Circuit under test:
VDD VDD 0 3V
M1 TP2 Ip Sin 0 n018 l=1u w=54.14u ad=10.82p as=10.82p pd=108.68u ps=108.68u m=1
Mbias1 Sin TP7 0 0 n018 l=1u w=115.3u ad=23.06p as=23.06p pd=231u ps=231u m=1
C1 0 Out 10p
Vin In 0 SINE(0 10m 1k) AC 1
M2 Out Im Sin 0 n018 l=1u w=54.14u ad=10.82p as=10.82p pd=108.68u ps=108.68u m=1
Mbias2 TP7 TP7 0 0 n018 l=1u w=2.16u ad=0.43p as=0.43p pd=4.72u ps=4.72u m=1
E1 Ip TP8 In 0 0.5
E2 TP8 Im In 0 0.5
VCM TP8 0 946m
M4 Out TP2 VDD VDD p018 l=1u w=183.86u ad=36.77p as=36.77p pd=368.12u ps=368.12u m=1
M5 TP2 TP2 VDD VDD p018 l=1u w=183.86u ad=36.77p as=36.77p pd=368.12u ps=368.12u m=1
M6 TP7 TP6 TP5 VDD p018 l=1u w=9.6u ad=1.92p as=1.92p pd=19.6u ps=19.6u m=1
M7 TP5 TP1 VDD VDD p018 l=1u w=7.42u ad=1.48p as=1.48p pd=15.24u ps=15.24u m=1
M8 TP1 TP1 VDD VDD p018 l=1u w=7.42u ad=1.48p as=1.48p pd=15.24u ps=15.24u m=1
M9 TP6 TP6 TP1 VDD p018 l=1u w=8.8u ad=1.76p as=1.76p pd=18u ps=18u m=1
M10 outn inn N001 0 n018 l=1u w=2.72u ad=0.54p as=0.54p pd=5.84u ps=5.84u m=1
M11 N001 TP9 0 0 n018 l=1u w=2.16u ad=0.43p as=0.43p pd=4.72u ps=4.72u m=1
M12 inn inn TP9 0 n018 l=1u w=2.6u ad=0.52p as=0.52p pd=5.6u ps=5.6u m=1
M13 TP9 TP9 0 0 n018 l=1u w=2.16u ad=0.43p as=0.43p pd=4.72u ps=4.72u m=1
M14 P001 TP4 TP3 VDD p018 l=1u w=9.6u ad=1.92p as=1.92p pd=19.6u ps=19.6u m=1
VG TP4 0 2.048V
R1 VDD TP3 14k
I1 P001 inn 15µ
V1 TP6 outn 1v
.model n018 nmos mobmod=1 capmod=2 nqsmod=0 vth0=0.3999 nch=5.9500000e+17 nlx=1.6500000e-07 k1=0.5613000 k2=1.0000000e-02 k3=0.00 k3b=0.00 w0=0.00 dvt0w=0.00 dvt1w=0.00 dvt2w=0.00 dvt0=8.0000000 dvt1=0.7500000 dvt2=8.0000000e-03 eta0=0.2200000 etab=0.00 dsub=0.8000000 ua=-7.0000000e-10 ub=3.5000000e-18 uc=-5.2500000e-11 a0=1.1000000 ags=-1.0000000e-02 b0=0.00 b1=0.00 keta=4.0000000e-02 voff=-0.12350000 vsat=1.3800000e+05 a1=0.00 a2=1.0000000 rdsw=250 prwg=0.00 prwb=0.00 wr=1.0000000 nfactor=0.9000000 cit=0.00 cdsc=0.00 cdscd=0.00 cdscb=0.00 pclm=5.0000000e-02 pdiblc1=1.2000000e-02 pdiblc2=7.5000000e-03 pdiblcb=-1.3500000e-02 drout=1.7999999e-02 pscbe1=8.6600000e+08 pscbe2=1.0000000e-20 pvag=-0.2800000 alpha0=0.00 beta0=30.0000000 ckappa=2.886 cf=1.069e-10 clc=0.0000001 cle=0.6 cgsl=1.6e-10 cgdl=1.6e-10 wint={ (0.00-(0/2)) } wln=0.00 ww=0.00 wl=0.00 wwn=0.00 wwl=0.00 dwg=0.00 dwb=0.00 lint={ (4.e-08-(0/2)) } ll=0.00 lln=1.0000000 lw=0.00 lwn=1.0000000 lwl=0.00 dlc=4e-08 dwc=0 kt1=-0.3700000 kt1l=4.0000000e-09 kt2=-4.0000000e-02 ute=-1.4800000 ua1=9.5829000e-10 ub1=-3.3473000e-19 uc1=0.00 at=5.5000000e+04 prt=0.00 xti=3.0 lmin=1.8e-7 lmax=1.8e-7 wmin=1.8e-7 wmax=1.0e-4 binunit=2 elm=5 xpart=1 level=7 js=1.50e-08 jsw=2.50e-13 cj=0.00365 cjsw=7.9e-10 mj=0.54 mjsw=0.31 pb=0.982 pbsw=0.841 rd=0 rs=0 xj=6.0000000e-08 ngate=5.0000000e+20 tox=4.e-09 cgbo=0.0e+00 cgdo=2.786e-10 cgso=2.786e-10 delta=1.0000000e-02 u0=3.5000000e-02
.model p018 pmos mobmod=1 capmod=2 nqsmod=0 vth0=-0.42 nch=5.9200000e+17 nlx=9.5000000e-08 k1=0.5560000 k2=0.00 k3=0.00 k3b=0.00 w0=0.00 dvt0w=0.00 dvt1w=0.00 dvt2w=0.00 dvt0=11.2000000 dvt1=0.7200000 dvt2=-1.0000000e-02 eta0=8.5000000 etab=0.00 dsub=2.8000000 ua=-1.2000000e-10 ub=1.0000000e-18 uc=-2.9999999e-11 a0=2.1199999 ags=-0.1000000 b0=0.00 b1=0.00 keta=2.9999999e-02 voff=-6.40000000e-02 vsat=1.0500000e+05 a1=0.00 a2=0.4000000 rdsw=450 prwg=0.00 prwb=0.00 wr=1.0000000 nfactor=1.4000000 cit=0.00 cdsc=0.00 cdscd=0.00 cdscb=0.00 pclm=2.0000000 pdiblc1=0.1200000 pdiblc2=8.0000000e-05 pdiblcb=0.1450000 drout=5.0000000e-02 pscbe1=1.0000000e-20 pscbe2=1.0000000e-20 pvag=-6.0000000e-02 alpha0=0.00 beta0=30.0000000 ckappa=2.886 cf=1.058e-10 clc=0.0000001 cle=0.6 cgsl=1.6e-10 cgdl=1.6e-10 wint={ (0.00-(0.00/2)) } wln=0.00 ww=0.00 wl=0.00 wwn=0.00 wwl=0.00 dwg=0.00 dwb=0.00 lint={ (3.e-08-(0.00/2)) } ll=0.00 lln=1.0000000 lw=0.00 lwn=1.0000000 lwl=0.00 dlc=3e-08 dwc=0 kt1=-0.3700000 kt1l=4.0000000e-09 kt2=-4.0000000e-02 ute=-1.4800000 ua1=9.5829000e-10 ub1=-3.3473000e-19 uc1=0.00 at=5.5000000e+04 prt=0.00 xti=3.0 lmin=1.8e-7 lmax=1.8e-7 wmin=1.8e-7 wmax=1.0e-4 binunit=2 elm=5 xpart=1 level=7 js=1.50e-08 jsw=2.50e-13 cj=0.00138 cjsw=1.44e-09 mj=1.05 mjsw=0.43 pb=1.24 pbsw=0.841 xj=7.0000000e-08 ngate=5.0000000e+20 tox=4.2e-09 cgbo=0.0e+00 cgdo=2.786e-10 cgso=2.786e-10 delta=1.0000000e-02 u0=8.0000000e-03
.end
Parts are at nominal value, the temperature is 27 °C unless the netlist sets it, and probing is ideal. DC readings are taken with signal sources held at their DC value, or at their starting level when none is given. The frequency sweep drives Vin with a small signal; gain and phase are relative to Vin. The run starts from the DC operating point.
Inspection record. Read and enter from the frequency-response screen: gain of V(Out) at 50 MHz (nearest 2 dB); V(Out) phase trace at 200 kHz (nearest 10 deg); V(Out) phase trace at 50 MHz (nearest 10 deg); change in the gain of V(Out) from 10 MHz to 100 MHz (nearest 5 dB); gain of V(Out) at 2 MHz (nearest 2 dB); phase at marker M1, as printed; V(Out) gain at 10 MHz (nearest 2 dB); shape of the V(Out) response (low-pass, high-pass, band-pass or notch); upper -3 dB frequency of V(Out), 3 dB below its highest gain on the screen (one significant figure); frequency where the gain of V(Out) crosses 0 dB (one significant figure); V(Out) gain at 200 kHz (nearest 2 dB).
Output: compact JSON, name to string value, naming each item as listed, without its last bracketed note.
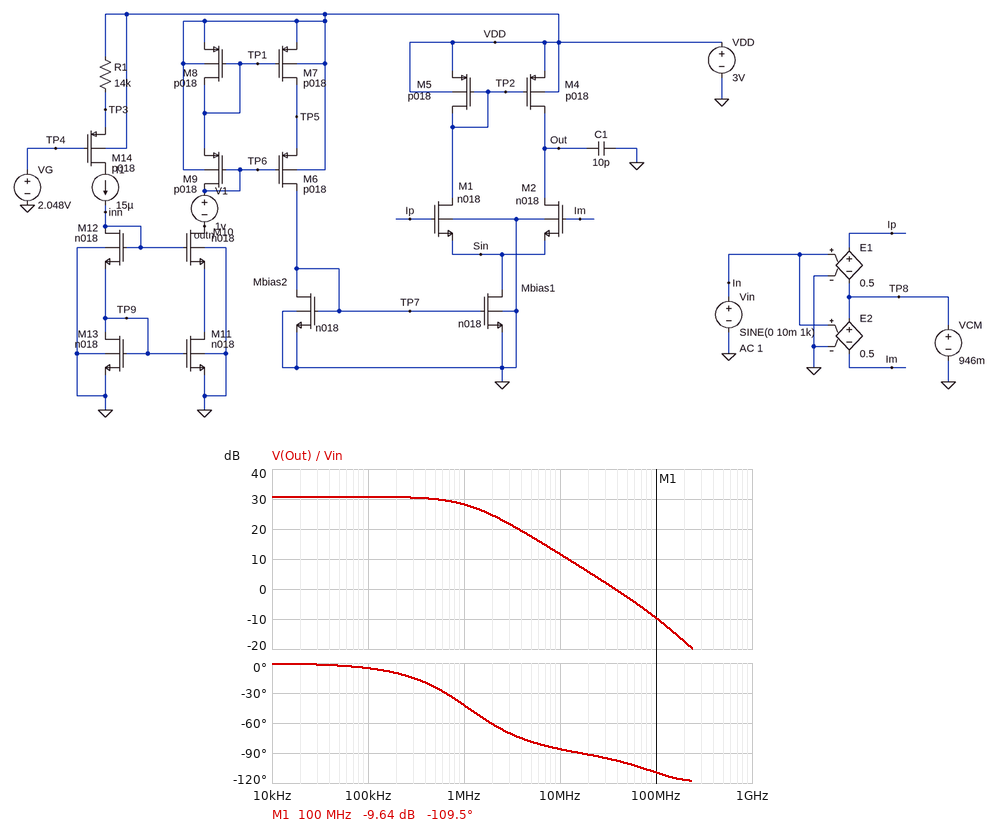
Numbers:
{"gain of V(Out) at 50 MHz": "-2 dB", "V(Out) phase trace at 200 kHz": "-10 deg", "V(Out) phase trace at 50 MHz": "-100 deg", "change in the gain of V(Out) from 10 MHz to 100 MHz": "-20 dB", "gain of V(Out) at 2 MHz": "24 dB", "phase at marker M1, as printed": "-109.5 deg", "V(Out) gain at 10 MHz": "12 dB", "shape of the V(Out) response": "low-pass", "upper -3 dB frequency of V(Out), 3 dB below its highest gain on the screen": "1 MHz", "frequency where the gain of V(Out) crosses 0 dB": "40 MHz", "V(Out) gain at 200 kHz": "30 dB"}
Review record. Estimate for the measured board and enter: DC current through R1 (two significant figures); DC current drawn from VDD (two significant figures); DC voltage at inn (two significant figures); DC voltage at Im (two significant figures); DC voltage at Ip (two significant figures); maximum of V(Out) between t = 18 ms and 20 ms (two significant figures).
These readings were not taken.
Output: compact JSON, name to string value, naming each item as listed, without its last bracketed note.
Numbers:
{"DC current through R1": "15 µA", "DC current drawn from VDD": "1.0 mA", "DC voltage at inn": "1.5 V", "DC voltage at Im": "950 mV", "DC voltage at Ip": "950 mV", "maximum of V(Out) between t = 18 ms and 20 ms": "2.5 V"}
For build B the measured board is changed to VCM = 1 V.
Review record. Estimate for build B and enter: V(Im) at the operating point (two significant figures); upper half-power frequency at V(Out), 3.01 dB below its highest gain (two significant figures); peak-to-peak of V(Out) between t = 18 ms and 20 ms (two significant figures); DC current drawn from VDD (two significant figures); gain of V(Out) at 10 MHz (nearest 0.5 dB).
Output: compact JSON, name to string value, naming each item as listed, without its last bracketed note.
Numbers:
{"V(Im) at the operating point": "1.0 V", "upper half-power frequency at V(Out), 3.01 dB below its highest gain": "1.0 MHz", "peak-to-peak of V(Out) between t = 18 ms and 20 ms": "920 mV", "DC current drawn from VDD": "1.1 mA", "gain of V(Out) at 10 MHz": "12.0 dB"}
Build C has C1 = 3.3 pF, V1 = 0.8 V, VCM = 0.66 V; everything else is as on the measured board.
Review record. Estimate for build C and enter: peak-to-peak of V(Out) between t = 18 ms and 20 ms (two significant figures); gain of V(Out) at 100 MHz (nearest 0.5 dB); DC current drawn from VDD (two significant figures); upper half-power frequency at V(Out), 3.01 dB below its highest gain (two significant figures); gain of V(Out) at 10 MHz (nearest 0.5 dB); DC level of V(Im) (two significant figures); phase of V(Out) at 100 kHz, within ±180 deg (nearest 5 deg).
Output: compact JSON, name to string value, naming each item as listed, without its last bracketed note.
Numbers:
{"peak-to-peak of V(Out) between t = 18 ms and 20 ms": "570 mV", "gain of V(Out) at 100 MHz": "-3.5 dB", "DC current drawn from VDD": "550 µA", "upper half-power frequency at V(Out), 3.01 dB below its highest gain": "3.2 MHz", "gain of V(Out) at 10 MHz": "18.0 dB", "DC level of V(Im)": "660 mV", "phase of V(Out) at 100 kHz, within ±180 deg": "0 deg"}
